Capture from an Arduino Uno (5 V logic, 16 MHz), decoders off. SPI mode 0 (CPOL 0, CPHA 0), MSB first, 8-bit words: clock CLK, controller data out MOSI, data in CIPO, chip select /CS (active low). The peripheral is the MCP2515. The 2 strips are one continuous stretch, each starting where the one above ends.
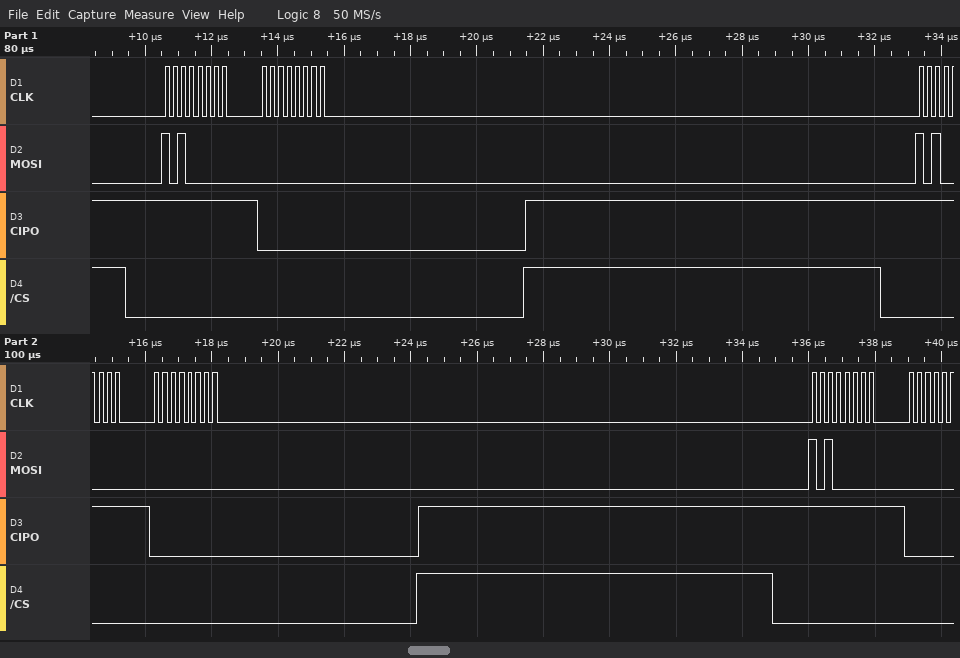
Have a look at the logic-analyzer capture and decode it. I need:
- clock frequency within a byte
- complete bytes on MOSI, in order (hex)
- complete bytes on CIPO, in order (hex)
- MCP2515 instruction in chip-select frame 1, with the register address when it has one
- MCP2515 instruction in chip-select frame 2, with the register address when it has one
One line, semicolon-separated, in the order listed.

4 MHz; A0 00 A0 00 A0; FF 00 FF 00 FF; READ STATUS; READ STATUS
